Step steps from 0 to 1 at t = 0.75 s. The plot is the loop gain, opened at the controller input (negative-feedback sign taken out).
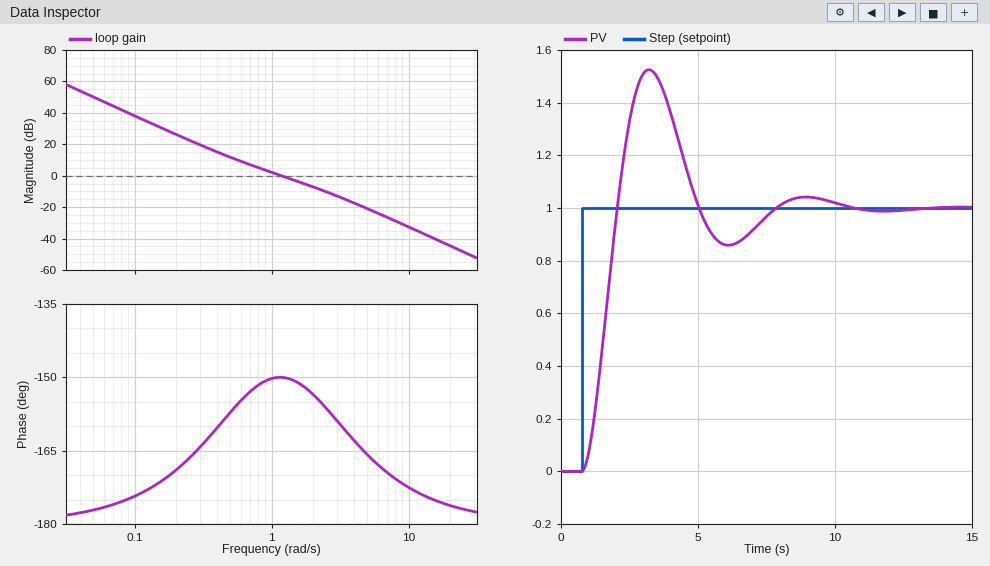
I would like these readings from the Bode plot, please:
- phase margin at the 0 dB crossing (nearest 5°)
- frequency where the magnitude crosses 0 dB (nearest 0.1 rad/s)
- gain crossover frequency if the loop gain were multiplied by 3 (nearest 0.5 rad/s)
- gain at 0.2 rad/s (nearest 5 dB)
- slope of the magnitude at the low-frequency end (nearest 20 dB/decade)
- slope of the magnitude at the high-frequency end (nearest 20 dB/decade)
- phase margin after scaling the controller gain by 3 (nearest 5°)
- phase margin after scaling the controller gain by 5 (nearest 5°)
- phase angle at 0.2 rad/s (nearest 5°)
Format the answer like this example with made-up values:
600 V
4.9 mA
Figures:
30°
1.2 rad/s
2.5 rad/s
25 dB
-40 dB/decade
-40 dB/decade
25°
20°
-170°
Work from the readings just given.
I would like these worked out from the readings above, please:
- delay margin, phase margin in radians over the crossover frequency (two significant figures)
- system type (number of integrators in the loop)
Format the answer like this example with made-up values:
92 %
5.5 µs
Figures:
0.44 s
2
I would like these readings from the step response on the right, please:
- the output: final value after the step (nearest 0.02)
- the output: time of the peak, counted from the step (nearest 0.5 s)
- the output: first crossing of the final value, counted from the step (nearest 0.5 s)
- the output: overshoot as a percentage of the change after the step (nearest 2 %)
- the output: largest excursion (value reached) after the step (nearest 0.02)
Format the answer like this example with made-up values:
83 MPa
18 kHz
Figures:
1.00
2.5 s
1.5 s
52 %
1.52
